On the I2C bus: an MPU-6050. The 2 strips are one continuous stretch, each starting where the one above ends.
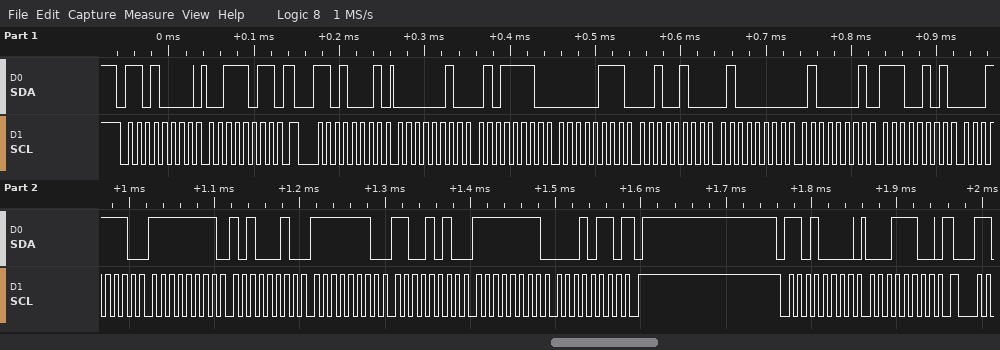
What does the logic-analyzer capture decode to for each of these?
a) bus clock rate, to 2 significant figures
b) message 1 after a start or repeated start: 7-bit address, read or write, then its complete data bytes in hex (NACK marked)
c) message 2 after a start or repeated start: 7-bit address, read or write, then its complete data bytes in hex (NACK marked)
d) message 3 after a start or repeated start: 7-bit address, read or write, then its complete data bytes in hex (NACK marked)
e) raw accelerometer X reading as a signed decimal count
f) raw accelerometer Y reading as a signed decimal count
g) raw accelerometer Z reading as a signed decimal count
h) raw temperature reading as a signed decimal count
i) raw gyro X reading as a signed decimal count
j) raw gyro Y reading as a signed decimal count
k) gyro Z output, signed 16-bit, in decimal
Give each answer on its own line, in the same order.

100 kHz
0x68 write: 3B
0x68 read: 02 5E 07 24 40 41 E5 1E FF A2 FE CA FF 16 NACK
0x68 write: 1C
606
1828
16449
-6882
-94
-310
-234
